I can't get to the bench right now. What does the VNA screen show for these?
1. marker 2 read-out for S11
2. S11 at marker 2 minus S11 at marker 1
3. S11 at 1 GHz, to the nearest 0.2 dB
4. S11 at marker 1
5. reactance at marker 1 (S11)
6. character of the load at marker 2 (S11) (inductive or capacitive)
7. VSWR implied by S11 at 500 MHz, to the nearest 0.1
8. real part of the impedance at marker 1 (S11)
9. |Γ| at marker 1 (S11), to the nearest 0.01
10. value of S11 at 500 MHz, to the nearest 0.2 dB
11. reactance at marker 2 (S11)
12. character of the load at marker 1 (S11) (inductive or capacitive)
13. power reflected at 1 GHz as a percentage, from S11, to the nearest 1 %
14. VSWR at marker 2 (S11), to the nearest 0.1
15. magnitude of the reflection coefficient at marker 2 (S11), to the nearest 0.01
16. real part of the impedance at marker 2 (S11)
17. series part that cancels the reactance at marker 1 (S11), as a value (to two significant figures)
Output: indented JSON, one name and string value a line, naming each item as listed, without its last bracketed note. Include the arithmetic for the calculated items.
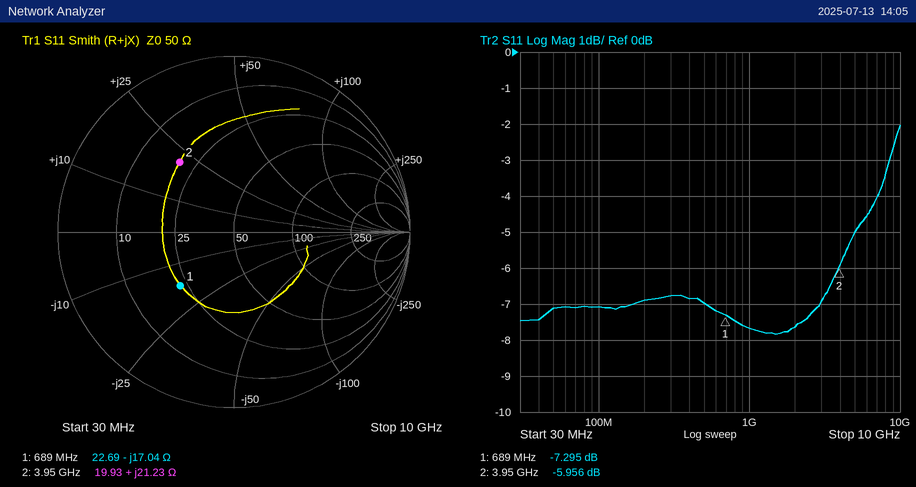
{
  "marker 2 read-out for S11": "-5.956 dB",
  "S11 at marker 2 minus S11 at marker 1": "-5.956 − (-7.295) = 1.339 dB",
  "S11 at 1 GHz, to the nearest 0.2 dB": "-7.6 dB",
  "S11 at marker 1": "-7.295 dB",
  "reactance at marker 1": "-17.04 Ω",
  "character of the load at marker 2 (S11)": "inductive",
  "VSWR implied by S11 at 500 MHz, to the nearest 0.1": "|Γ| = 10^(-7/20) = 0.4467; VSWR = (1 + 0.4467)/(1 − 0.4467) ≈ 2.6",
  "real part of the impedance at marker 1": "22.69 Ω",
  "|Γ| at marker 1 (S11), to the nearest 0.01": "0.43",
  "value of S11 at 500 MHz, to the nearest 0.2 dB": "-7.0 dB",
  "reactance at marker 2": "+21.23 Ω",
  "character of the load at marker 1 (S11)": "capacitive",
  "power reflected at 1 GHz as a percentage, from S11, to the nearest 1 %": "10^(-7.6/10) ≈ 17 %",
  "VSWR at marker 2 (S11), to the nearest 0.1": "3.0",
  "magnitude of the reflection coefficient at marker 2 (S11), to the nearest 0.01": "10^(-5.956/20) ≈ 0.50",
  "real part of the impedance at marker 2": "19.93 Ω",
  "series part that cancels the reactance at marker 1 (S11), as a value": "L = 17.04 Ω/(2π × 689 MHz) ≈ 3.9 nH"
}
